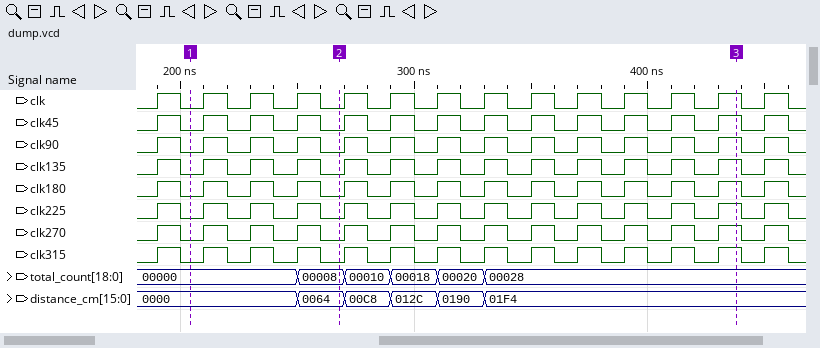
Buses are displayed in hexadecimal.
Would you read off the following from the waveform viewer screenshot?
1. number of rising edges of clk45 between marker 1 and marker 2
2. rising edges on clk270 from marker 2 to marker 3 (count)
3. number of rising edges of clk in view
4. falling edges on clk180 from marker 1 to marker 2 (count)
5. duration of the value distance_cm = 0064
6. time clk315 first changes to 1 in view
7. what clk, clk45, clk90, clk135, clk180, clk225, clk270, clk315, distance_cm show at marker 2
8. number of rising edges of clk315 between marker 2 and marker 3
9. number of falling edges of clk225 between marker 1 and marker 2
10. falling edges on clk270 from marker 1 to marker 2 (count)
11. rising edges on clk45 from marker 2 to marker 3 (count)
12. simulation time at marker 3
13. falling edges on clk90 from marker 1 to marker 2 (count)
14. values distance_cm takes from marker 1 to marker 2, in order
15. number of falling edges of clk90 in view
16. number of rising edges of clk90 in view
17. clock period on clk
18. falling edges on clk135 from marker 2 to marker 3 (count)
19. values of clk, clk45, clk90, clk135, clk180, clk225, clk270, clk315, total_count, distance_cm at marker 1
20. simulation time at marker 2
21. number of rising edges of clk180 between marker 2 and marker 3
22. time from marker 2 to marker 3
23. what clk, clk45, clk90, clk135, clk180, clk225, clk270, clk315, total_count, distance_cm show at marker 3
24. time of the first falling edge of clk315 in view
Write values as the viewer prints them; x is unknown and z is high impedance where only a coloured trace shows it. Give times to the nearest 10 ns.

3
9
14
3
20 ns
190 ns
clk=0, clk45=0, clk90=0, clk135=0, clk180=0, clk225=0, clk270=0, clk315=0, distance_cm=0064
9
3
3
9
440 ns
3
0000, 0064
14
14
20 ns
8
clk=0, clk45=0, clk90=0, clk135=0, clk180=0, clk225=0, clk270=0, clk315=0, total_count=00000, distance_cm=0000
270 ns
9
170 ns
clk=1, clk45=1, clk90=1, clk135=1, clk180=1, clk225=1, clk270=1, clk315=1, total_count=00028, distance_cm=01F4
200 ns
